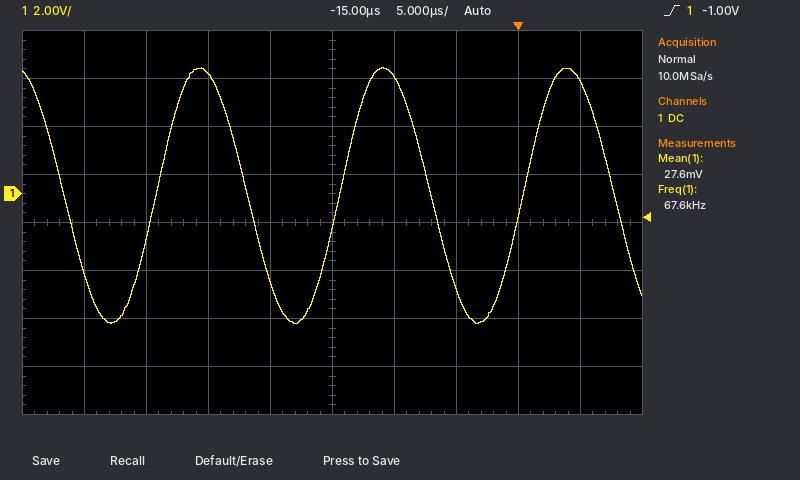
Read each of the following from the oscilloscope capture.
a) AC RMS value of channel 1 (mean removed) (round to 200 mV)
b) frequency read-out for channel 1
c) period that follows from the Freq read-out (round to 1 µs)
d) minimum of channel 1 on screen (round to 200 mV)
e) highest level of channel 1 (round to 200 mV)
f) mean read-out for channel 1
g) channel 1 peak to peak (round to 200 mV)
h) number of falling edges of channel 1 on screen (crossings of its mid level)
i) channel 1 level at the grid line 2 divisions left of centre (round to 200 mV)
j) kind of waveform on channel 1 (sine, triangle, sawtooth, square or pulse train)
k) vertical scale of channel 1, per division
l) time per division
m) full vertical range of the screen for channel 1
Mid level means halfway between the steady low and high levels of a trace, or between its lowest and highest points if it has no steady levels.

3.8 V
67.6 kHz
15 µs
-5.4 V
5.2 V
27.6 mV
10.6 V
4
5.0 V
sine
2 V
5 µs
16 V
